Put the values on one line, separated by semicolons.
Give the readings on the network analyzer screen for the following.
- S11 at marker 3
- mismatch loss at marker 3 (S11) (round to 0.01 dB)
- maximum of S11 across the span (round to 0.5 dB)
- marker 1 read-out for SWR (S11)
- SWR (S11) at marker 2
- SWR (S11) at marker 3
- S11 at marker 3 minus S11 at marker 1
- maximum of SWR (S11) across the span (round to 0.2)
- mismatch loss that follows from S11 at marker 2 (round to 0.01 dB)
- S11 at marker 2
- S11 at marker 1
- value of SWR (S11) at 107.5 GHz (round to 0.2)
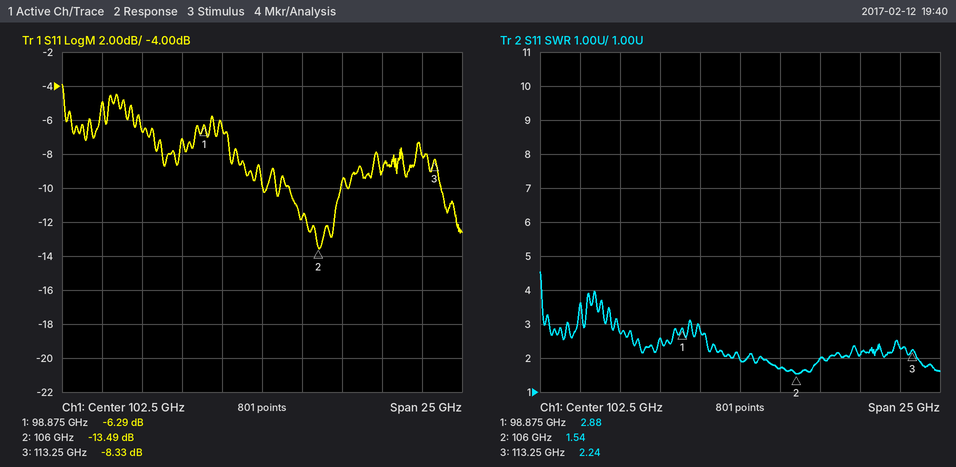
-8.33 dB; 0.69 dB; -4.0 dB; 2.88; 1.54; 2.24; -2.04 dB; 4.6; 0.20 dB; -13.49 dB; -6.29 dB; 2.0
